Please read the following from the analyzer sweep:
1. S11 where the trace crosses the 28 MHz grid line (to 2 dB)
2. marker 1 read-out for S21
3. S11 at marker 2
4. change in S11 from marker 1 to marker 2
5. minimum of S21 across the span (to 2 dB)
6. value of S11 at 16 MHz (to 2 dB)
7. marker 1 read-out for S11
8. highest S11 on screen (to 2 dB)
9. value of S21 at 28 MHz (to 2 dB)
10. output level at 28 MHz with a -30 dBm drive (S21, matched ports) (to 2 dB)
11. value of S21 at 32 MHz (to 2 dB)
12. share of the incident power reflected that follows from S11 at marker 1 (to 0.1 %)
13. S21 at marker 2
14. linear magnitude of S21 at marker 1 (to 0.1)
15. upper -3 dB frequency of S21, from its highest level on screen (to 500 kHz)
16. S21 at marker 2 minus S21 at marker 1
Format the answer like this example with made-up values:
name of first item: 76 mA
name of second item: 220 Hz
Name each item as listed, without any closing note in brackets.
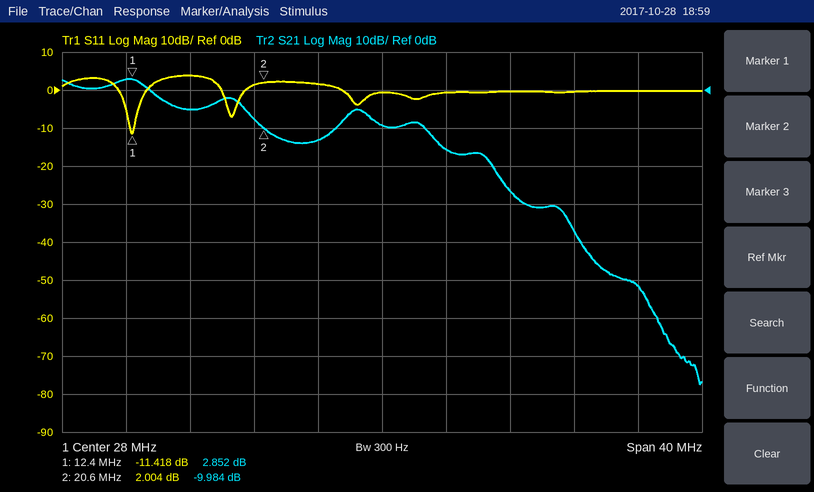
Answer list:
S11 where the trace crosses the 28 MHz grid line: 0 dB
marker 1 read-out for S21: 2.852 dB
S11 at marker 2: 2.004 dB
change in S11 from marker 1 to marker 2: 13.422 dB
minimum of S21 across the span: -78 dB
value of S11 at 16 MHz: 4 dB
marker 1 read-out for S11: -11.418 dB
highest S11 on screen: 4 dB
value of S21 at 28 MHz: -10 dB
output level at 28 MHz with a -30 dBm drive (S21, matched ports): -40 dBm
value of S21 at 32 MHz: -16 dB
share of the incident power reflected that follows from S11 at marker 1: 7.2 %
S21 at marker 2: -9.984 dB
linear magnitude of S21 at marker 1: 1.4
upper -3 dB frequency of S21, from its highest level on screen: 13.5 MHz
S21 at marker 2 minus S21 at marker 1: -12.836 dB
